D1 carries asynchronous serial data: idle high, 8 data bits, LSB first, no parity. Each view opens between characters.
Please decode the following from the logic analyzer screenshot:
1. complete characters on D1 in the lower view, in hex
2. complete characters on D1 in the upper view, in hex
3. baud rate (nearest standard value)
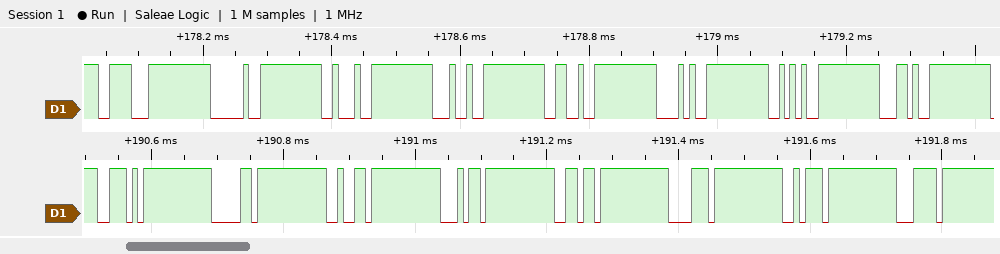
AE, B0, B2, B4, B6, B8, BA, BC
1E, 20, 22, 24, 26, 28, 2A, 2C
115200 baud
